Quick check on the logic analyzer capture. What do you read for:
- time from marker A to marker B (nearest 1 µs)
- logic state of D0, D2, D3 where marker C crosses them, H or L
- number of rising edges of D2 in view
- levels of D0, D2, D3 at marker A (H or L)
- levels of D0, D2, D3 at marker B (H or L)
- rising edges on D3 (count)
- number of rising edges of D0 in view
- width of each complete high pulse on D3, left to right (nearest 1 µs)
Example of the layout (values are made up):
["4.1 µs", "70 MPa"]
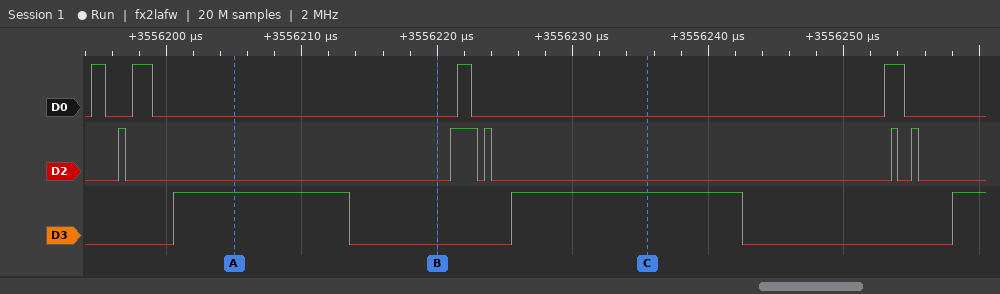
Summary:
["15 µs", "D0=L, D2=L, D3=H", "5", "D0=L, D2=L, D3=H", "D0=L, D2=L, D3=L", "3", "4", "13 µs, 17 µs"]
